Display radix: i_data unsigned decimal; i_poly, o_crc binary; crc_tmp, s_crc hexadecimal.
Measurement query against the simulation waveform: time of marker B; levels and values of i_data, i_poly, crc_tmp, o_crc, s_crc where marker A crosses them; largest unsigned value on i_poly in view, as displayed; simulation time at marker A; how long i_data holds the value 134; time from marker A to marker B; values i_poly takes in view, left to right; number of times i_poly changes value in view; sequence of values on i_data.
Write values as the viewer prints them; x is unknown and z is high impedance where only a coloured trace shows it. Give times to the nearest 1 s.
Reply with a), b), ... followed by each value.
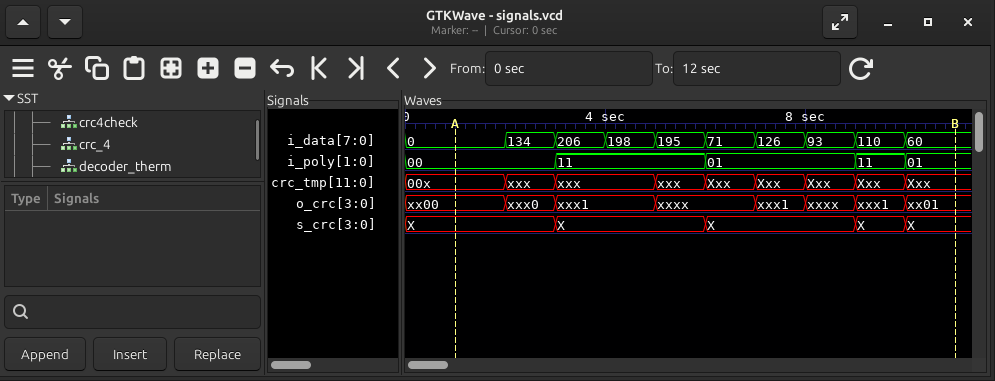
a) 11 s
b) i_data=0, i_poly=00, crc_tmp=00x, o_crc=xx00, s_crc=X
c) 11
d) 1 s
e) 1 s
f) 10 s
g) 00, 11, 01, 11, 01
h) 4
i) 0, 134, 206, 198, 195, 71, 126, 93, 110, 60
